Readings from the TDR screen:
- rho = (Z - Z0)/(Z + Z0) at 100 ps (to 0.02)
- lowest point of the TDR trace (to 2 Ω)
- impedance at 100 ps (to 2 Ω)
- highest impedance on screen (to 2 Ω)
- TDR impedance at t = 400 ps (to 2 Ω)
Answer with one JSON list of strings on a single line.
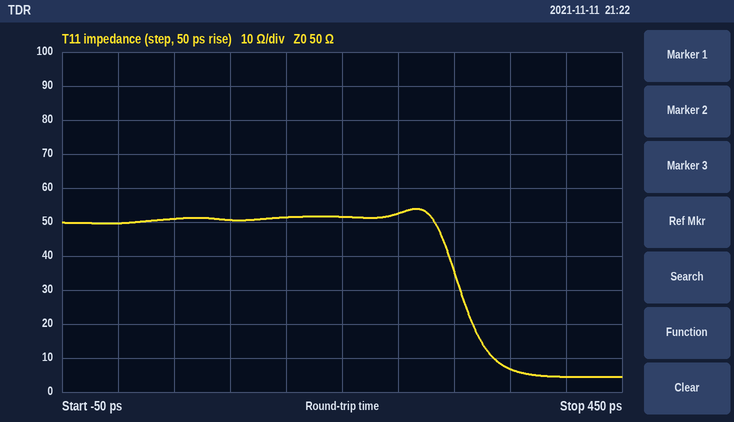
["0.00", "4 Ω", "50 Ω", "54 Ω", "4 Ω"]
